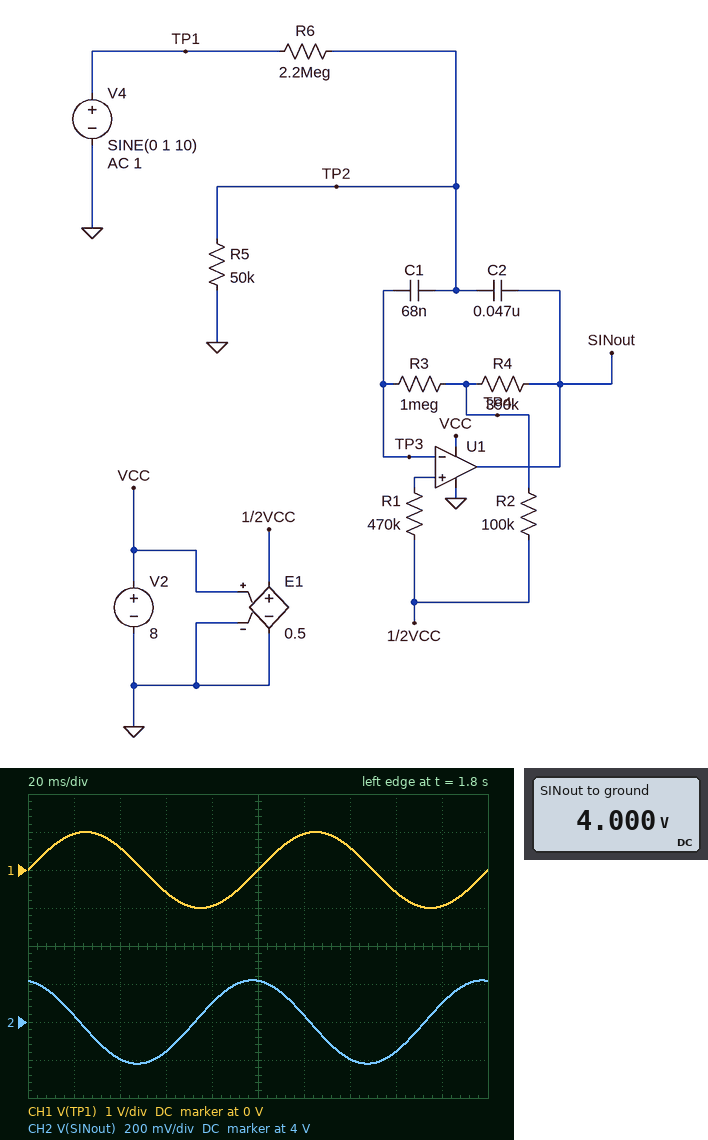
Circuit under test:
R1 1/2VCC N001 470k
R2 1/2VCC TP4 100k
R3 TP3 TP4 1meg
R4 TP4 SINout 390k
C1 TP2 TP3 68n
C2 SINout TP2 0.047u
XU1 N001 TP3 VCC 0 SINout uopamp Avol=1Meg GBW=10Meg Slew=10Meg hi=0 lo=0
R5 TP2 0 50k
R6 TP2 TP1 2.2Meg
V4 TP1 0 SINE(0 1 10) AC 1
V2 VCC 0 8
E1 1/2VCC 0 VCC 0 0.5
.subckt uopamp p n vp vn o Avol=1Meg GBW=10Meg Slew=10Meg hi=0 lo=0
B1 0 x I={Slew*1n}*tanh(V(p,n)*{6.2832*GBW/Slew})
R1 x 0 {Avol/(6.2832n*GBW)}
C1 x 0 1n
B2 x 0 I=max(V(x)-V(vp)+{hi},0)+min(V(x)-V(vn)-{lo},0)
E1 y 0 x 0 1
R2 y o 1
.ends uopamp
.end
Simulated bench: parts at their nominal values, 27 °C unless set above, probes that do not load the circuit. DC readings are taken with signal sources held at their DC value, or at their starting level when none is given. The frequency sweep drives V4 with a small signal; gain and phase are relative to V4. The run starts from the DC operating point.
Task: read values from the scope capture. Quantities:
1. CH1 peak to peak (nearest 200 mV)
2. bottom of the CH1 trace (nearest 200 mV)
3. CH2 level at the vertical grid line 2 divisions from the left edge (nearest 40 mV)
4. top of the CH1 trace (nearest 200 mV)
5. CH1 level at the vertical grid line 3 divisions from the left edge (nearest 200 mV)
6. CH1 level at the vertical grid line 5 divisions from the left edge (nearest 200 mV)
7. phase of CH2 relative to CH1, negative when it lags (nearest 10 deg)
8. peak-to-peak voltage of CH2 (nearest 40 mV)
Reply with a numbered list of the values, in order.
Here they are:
1. 2.0 V
2. -1.0 V
3. 3.80 V
4. 1.0 V
5. -600 mV
6. 0 V
7. 100 deg
8. 440 mV
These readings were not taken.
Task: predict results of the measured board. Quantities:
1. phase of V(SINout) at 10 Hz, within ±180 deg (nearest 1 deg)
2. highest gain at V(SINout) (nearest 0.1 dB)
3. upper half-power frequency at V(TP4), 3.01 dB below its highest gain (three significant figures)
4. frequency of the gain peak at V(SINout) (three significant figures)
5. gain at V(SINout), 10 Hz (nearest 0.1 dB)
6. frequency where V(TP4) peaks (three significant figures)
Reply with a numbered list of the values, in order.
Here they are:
1. 99 deg
2. 3.1 dB
3. 6.10 Hz
4. 5.54 Hz
5. -13.2 dB
6. 5.54 Hz
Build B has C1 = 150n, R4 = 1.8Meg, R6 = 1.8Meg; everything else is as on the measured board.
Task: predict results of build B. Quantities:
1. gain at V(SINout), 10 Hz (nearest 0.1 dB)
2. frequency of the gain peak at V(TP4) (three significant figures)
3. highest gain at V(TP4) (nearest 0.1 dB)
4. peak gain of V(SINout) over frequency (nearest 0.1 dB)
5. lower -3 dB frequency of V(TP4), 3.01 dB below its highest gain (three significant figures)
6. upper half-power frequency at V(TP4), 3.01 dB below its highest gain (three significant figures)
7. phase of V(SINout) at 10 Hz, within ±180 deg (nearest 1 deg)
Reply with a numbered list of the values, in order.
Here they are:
1. -14.2 dB
2. 1.88 Hz
3. -7.5 dB
4. 18.9 dB
5. 1.78 Hz
6. 1.99 Hz
7. 91 deg
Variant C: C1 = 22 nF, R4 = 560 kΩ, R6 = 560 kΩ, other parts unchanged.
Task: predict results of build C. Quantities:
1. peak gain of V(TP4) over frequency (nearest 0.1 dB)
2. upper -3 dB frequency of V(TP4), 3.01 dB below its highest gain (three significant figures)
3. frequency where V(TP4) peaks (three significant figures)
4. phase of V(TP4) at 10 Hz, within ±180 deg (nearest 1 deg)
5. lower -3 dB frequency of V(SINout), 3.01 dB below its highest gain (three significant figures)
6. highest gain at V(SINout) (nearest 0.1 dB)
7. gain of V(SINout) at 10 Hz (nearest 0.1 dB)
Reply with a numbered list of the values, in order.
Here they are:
1. -4.9 dB
2. 9.41 Hz
3. 8.63 Hz
4. 120 deg
5. 7.92 Hz
6. 12.2 dB
7. 6.2 dB
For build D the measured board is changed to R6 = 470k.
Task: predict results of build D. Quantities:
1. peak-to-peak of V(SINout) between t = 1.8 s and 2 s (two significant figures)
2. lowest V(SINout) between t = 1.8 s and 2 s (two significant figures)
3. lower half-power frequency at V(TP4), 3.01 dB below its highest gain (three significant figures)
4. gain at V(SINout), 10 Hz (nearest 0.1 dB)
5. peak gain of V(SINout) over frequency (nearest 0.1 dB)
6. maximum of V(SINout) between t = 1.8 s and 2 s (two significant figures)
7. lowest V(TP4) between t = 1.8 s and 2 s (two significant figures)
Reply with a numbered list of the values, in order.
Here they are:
1. 2.1 V
2. 2.9 V
3. 5.24 Hz
4. 0.5 dB
5. 16.5 dB
6. 5.1 V
7. 3.8 V
